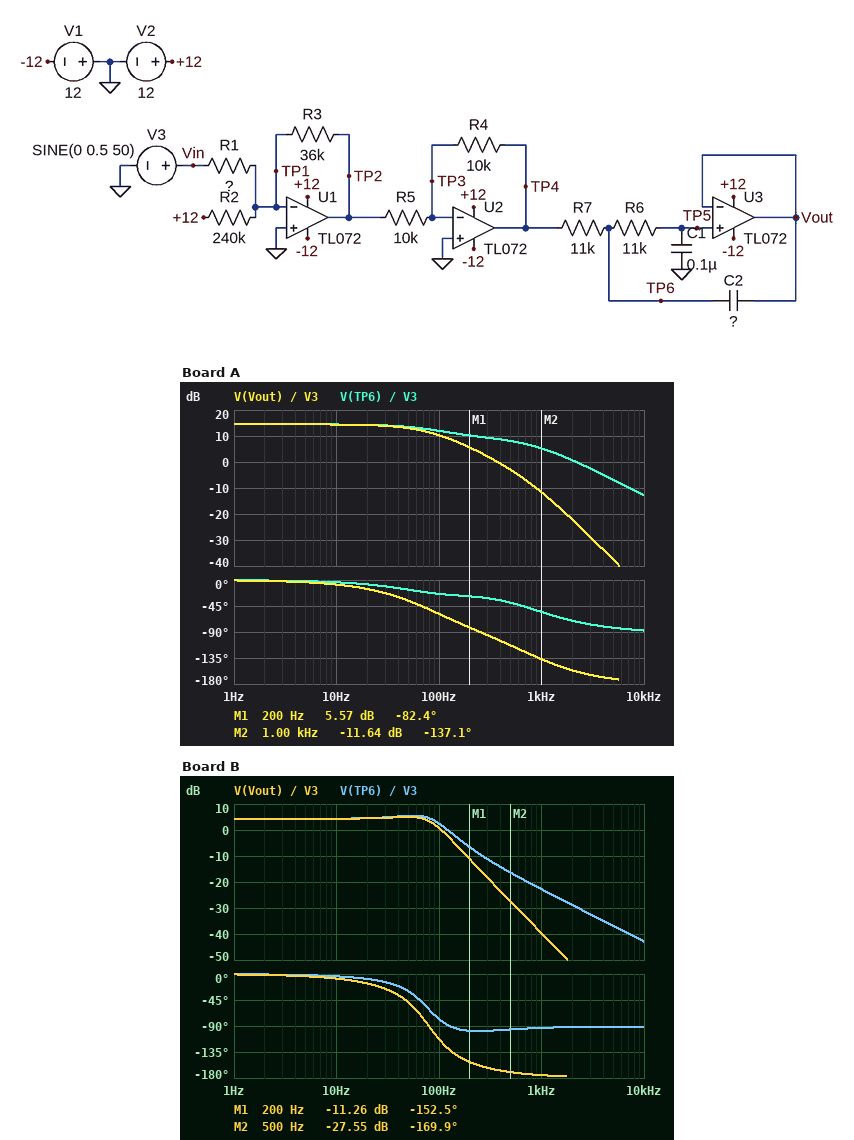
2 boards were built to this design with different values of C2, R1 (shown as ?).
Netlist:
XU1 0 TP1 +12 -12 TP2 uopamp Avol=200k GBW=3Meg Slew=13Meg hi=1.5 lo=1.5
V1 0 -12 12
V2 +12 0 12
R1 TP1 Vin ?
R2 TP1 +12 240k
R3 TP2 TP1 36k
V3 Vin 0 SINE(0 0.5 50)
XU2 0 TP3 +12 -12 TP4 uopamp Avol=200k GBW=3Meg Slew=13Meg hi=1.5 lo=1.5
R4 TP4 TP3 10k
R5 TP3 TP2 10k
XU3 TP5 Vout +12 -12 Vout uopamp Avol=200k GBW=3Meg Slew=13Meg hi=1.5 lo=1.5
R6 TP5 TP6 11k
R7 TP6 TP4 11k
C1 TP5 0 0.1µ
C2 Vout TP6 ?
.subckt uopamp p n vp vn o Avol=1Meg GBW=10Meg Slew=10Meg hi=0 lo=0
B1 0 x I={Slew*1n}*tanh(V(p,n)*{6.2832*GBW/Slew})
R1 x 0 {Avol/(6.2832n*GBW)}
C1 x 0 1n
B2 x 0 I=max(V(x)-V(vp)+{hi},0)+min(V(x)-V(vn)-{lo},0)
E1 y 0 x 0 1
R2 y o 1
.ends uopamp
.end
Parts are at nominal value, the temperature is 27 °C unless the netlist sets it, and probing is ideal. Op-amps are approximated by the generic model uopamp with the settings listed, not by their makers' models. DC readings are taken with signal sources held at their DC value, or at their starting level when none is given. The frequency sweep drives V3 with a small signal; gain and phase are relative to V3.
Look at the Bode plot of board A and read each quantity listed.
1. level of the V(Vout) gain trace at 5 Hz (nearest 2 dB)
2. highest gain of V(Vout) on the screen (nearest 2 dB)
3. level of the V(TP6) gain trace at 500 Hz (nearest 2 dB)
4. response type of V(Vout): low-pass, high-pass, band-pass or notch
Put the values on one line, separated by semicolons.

14 dB; 14 dB; 8 dB; low-pass
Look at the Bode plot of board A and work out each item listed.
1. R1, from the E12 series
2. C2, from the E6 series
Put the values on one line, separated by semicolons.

6.8 kΩ; 33 nF
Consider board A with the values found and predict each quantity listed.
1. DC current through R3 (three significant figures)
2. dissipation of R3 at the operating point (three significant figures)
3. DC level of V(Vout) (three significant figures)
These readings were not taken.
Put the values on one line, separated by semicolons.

50.0 µA; 90.0 µW; 1.80 V
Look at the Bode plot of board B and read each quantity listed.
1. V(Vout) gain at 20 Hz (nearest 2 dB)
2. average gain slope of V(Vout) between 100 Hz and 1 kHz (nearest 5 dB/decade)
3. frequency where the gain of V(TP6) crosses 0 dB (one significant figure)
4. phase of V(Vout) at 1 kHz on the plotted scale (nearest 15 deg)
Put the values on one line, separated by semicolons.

4 dB; -40 dB/decade; 100 Hz; -180 deg
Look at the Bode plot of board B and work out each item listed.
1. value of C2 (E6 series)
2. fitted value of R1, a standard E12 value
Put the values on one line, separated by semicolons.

330 nF; 22 kΩ
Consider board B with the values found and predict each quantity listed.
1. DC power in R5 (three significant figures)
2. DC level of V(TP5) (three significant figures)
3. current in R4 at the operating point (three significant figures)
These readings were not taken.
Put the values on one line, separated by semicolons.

324 µW; 1.80 V; 180 µA
